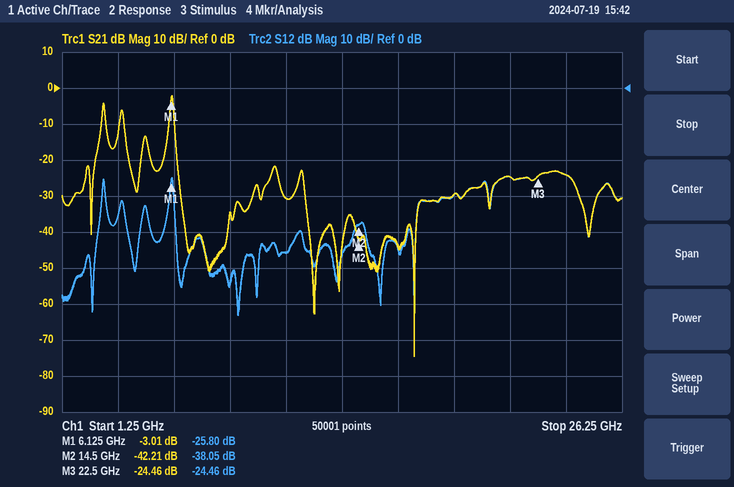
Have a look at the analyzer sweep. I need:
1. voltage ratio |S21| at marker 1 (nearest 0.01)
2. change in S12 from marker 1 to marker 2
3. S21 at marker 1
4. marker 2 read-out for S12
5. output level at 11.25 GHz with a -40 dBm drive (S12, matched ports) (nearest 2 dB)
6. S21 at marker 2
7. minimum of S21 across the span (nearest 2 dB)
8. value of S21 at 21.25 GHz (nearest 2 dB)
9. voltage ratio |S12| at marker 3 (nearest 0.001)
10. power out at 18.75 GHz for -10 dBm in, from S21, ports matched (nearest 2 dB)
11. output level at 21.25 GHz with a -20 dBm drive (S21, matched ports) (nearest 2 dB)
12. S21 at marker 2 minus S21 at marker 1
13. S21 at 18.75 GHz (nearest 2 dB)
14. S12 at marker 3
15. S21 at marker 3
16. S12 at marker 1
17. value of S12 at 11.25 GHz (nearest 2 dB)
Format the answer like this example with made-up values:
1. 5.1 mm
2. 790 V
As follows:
1. 0.71
2. -12.25 dB
3. -3.01 dB
4. -38.05 dB
5. -86 dBm
6. -42.21 dB
7. -74 dB
8. -24 dB
9. 0.060
10. -40 dBm
11. -44 dBm
12. -39.20 dB
13. -30 dB
14. -24.46 dB
15. -24.46 dB
16. -25.80 dB
17. -46 dB
